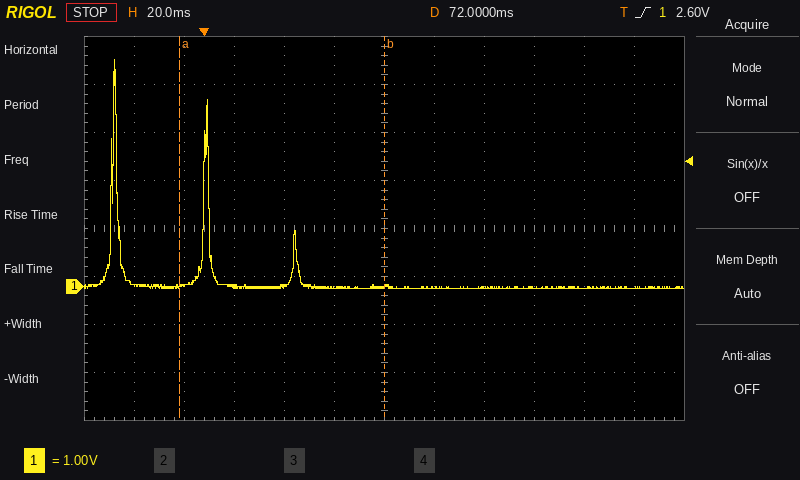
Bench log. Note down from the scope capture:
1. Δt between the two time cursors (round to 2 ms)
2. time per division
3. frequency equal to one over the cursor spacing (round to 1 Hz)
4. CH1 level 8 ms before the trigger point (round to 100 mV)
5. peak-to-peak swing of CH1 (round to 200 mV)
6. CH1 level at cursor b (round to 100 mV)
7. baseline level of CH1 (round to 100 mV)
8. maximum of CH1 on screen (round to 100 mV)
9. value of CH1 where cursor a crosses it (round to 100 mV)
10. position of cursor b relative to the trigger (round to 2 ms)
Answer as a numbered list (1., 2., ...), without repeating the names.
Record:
1. 82 ms
2. 20 ms
3. 12 Hz
4. 0.0 V
5. 4.8 V
6. 0.0 V
7. 0.0 V
8. 4.7 V
9. 0.0 V
10. +72 ms
